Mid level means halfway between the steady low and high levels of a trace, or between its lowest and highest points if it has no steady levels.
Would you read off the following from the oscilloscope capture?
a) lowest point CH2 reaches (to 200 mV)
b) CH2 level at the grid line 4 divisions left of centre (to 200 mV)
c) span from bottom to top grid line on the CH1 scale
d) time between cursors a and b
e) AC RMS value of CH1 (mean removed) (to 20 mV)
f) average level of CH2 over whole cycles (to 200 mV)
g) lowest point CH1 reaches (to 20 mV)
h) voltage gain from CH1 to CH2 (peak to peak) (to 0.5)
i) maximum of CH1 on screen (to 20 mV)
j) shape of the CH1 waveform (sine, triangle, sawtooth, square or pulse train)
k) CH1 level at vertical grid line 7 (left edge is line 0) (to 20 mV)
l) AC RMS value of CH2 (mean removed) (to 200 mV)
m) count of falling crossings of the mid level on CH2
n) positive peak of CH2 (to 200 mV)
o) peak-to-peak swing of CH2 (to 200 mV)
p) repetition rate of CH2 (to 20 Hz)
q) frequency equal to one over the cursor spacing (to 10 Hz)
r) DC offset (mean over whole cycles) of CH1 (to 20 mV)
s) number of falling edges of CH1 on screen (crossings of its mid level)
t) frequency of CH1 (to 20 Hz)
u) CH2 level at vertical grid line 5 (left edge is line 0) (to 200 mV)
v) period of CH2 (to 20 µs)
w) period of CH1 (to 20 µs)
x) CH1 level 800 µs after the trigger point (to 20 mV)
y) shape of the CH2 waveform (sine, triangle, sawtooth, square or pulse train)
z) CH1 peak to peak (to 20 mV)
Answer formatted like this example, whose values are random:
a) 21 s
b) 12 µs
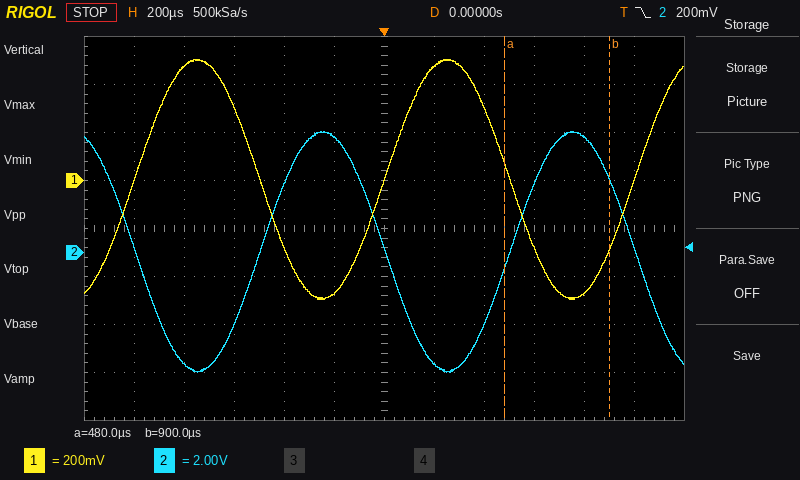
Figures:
a) -5.0 V
b) -4.6 V
c) 1.6 V
d) 420 µs
e) 360 mV
f) 0.0 V
g) -500 mV
h) 10.0
i) 500 mV
j) sine
k) 480 mV
l) 3.6 V
m) 3
n) 5.0 V
o) 10.0 V
p) 1.00 kHz
q) 2.38 kHz
r) 0 mV
s) 2
t) 1.00 kHz
u) 4.8 V
v) 1.00 ms
w) 1.00 ms
x) -460 mV
y) sine
z) 1.00 V
